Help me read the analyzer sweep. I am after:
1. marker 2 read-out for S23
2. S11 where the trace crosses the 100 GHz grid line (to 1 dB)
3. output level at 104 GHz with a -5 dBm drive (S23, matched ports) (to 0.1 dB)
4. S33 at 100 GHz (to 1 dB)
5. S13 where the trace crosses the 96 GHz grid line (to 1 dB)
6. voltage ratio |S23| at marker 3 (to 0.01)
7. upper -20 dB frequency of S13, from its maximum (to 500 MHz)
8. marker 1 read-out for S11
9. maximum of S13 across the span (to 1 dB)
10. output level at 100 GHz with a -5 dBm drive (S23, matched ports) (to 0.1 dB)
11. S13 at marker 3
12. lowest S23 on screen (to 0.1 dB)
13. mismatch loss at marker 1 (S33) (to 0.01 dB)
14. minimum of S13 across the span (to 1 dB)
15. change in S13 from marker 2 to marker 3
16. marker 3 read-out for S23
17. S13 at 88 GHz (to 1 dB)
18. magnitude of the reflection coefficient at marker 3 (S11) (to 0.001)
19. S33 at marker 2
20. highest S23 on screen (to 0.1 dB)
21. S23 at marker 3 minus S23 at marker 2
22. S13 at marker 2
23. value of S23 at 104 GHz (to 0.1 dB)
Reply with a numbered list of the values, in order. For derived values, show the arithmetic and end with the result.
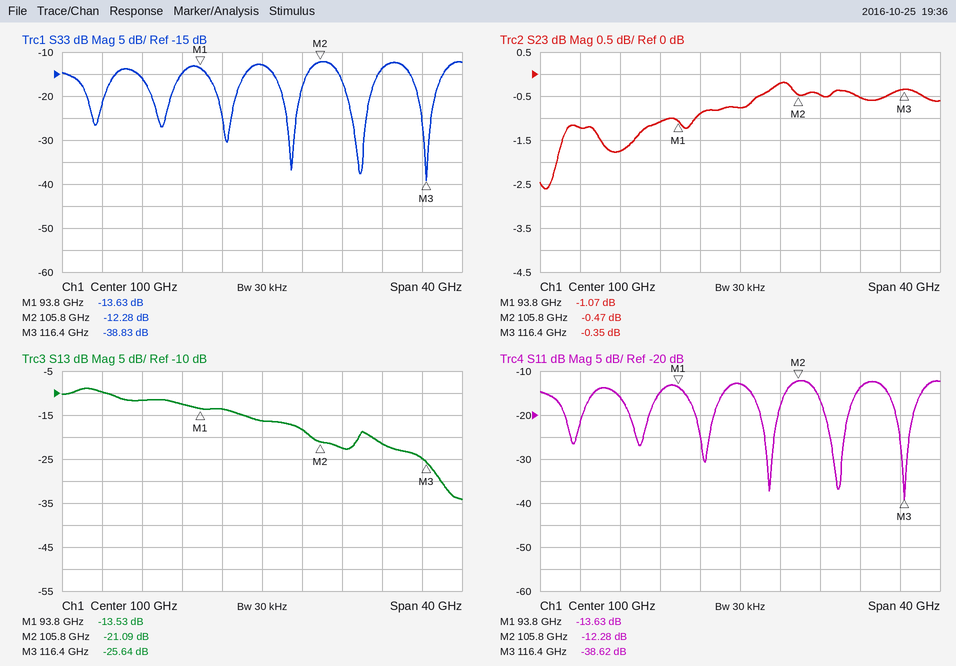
1. -0.47 dB
2. -13 dB
3. -5 dBm + (-0.2 dB) = -5.2 dBm
4. -13 dB
5. -14 dB
6. 10^(-0.35/20) ≈ 0.96
7. 117.5 GHz
8. -13.63 dB
9. -9 dB
10. -5 dBm + (-0.8 dB) = -5.8 dBm
11. -25.64 dB
12. -2.6 dB
13. −10 log10(1 − 10^(-13.63/10)) ≈ 0.19 dB
14. -34 dB
15. -25.64 − (-21.09) = -4.55 dB
16. -0.35 dB
17. -12 dB
18. 10^(-38.62/20) ≈ 0.012
19. -12.28 dB
20. -0.2 dB
21. -0.35 − (-0.47) = 0.12 dB
22. -21.09 dB
23. -0.2 dB
